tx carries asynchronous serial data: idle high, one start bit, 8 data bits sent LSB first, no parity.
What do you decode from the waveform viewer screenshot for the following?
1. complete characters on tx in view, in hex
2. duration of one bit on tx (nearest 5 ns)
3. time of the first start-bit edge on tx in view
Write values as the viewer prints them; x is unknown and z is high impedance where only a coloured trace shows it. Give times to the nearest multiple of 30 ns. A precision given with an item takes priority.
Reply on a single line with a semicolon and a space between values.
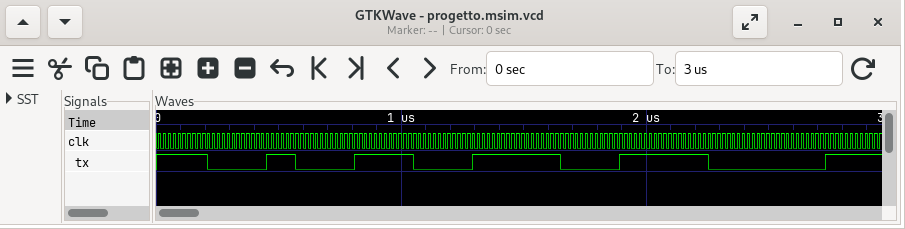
32, 0E; 120 ns; 210 ns
